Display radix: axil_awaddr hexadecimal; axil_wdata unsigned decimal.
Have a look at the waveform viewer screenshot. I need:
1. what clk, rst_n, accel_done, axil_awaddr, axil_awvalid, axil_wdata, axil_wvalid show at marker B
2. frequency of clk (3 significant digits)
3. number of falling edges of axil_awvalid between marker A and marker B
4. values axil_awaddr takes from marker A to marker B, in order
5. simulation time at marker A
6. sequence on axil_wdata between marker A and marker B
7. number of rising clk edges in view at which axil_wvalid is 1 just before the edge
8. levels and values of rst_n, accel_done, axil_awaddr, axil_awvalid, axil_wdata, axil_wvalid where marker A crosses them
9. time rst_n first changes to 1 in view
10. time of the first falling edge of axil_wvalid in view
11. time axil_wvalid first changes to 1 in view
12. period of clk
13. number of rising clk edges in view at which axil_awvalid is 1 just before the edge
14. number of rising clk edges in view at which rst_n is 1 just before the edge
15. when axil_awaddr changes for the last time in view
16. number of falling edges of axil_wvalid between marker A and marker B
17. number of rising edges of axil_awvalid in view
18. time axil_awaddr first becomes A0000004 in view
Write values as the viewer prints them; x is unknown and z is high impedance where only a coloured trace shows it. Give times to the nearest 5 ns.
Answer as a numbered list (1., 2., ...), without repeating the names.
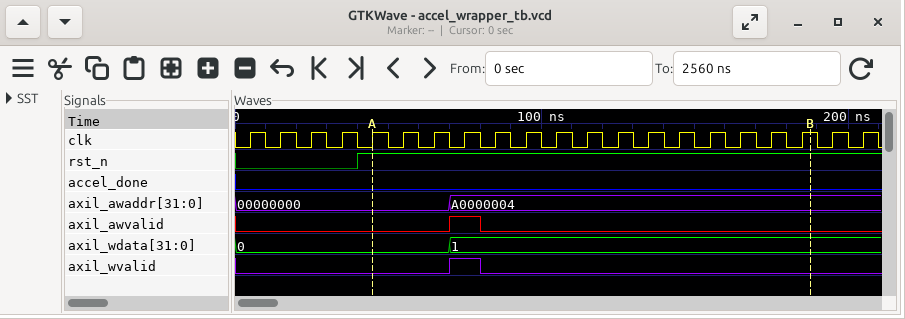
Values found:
1. clk=1, rst_n=1, accel_done=0, axil_awaddr=A0000004, axil_awvalid=0, axil_wdata=1, axil_wvalid=0
2. 100 MHz
3. 1
4. 00000000, A0000004
5. 45 ns
6. 0, 1
7. 1
8. rst_n=1, accel_done=0, axil_awaddr=00000000, axil_awvalid=0, axil_wdata=0, axil_wvalid=0
9. 40 ns
10. 80 ns
11. 70 ns
12. 10 ns
13. 1
14. 17
15. 70 ns
16. 1
17. 1
18. 70 ns
